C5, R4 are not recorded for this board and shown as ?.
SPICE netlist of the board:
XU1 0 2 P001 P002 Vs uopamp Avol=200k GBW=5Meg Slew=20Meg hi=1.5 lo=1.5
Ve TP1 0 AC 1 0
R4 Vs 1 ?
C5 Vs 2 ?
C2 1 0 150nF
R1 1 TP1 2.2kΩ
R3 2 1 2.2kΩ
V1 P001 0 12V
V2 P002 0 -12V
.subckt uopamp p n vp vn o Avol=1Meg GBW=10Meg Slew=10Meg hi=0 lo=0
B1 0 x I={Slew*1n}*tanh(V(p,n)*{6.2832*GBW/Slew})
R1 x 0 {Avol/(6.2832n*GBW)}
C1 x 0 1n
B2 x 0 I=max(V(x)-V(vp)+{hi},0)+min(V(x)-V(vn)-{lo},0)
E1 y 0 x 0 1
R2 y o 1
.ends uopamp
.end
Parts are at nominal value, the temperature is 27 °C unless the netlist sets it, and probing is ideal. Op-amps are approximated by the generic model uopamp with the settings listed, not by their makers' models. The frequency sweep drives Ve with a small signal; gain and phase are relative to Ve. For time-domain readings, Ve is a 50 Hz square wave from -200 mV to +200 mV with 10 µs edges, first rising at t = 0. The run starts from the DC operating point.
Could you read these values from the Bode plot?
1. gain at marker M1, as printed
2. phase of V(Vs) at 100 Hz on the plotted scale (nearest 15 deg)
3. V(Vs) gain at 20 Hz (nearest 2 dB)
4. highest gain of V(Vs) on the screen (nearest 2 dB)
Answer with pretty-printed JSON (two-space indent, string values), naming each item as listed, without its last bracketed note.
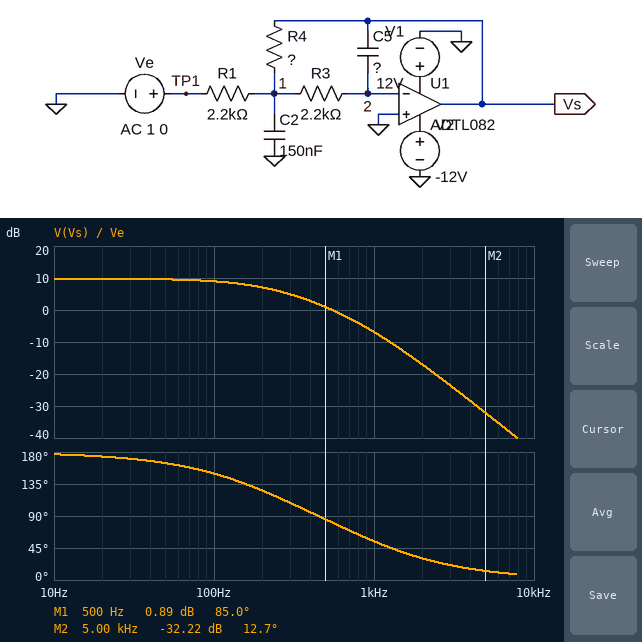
{
  "gain at marker M1, as printed": "0.89 dB",
  "phase of V(Vs) at 100 Hz on the plotted scale": "150 deg",
  "V(Vs) gain at 20 Hz": "10 dB",
  "highest gain of V(Vs) on the screen": "10 dB"
}
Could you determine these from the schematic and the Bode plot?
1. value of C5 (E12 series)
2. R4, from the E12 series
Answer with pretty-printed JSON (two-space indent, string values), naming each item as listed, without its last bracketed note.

{
  "value of C5": "56 nF",
  "R4, from the E12 series": "6.8 kΩ"
}
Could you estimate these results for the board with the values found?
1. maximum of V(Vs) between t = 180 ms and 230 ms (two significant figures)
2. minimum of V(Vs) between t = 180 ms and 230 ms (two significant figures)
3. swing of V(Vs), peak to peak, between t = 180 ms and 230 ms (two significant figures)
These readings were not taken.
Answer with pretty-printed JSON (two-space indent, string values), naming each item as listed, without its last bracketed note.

{
  "maximum of V(Vs) between t = 180 ms and 230 ms": "620 mV",
  "minimum of V(Vs) between t = 180 ms and 230 ms": "-620 mV",
  "swing of V(Vs), peak to peak, between t = 180 ms and 230 ms": "1.2 V"
}
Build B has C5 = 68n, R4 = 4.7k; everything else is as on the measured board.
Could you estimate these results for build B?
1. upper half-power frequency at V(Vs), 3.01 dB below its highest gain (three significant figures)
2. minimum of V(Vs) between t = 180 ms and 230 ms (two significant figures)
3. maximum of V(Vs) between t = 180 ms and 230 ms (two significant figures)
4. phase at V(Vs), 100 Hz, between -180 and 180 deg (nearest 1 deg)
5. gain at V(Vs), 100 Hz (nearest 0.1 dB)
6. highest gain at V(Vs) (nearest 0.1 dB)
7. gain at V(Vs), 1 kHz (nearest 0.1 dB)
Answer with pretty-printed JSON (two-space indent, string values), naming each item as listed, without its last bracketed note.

{
  "upper half-power frequency at V(Vs), 3.01 dB below its highest gain": "241 Hz",
  "minimum of V(Vs) between t = 180 ms and 230 ms": "-430 mV",
  "maximum of V(Vs) between t = 180 ms and 230 ms": "430 mV",
  "phase at V(Vs), 100 Hz, between -180 and 180 deg": "153 deg",
  "gain at V(Vs), 100 Hz": "5.9 dB",
  "highest gain at V(Vs)": "6.6 dB",
  "gain at V(Vs), 1 kHz": "-8.8 dB"
}
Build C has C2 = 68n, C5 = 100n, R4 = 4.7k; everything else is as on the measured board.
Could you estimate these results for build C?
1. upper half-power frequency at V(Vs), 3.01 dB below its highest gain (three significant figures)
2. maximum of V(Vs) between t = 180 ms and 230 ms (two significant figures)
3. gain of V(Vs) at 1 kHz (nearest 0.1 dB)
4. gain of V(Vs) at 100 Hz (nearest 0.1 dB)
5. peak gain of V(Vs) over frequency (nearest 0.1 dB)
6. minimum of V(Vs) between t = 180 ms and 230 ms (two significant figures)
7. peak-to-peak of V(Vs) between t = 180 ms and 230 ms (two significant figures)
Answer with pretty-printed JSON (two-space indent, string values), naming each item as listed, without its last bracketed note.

{
  "upper half-power frequency at V(Vs), 3.01 dB below its highest gain": "145 Hz",
  "maximum of V(Vs) between t = 180 ms and 230 ms": "430 mV",
  "gain of V(Vs) at 1 kHz": "-10.9 dB",
  "gain of V(Vs) at 100 Hz": "4.9 dB",
  "peak gain of V(Vs) over frequency": "6.6 dB",
  "minimum of V(Vs) between t = 180 ms and 230 ms": "-430 mV",
  "peak-to-peak of V(Vs) between t = 180 ms and 230 ms": "850 mV"
}
